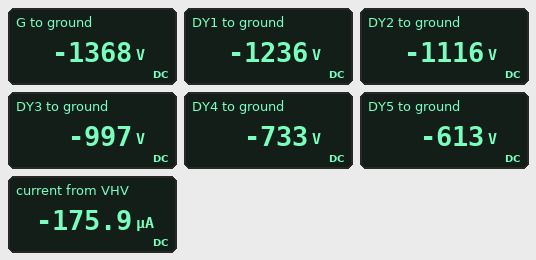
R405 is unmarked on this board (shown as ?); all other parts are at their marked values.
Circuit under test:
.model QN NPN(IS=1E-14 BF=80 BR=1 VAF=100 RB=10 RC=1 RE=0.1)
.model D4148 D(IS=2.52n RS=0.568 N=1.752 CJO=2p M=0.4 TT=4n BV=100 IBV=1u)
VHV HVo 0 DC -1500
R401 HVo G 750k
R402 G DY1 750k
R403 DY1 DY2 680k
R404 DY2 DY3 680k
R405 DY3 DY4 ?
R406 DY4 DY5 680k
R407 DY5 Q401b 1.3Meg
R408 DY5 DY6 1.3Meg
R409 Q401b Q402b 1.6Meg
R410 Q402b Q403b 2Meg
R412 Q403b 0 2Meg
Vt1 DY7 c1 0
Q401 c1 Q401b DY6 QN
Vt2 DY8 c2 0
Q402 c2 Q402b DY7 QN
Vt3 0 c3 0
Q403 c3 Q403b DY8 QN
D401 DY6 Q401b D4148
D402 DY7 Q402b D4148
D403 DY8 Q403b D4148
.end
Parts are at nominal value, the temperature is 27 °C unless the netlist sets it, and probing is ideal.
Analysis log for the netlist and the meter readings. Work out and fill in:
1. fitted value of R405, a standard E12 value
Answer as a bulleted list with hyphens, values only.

- 1.5 MΩ
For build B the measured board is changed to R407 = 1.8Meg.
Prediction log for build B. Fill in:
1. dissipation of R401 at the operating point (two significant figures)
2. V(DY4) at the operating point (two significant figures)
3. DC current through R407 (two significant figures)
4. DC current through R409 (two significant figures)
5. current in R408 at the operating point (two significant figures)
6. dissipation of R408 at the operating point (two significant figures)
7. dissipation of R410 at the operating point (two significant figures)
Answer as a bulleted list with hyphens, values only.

- 25 mW
- -700 V
- 77 µA
- 78 µA
- 110 µA
- 15 mW
- 12 mW
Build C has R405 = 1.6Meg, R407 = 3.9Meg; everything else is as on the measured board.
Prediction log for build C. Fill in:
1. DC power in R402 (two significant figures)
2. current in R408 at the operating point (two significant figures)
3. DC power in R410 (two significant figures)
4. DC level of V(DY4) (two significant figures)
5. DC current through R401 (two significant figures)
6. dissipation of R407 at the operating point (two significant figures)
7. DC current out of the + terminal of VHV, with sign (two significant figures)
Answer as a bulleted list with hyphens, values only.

- 29 mW
- 150 µA
- 5.3 mW
- -620 V
- 200 µA
- 9.6 mW
- -200 µA
